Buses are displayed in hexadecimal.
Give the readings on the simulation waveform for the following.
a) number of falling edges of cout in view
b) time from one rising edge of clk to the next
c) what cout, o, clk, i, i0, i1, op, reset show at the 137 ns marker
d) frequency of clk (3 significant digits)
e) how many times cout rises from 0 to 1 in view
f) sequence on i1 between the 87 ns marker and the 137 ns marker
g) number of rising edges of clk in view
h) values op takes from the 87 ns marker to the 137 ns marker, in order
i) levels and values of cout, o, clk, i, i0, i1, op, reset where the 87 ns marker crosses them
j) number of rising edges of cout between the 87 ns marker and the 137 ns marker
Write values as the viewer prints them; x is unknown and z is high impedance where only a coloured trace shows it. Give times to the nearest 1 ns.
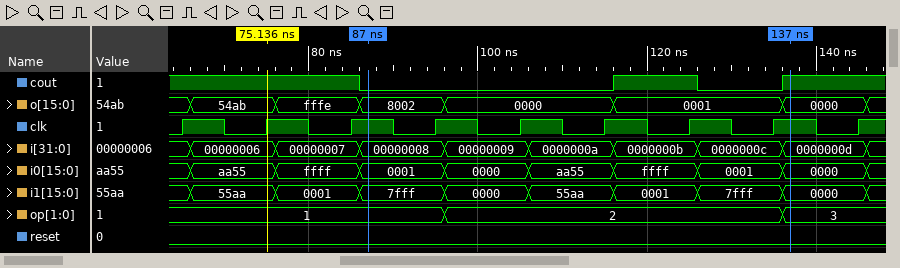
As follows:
2
10 ns
cout=1, o=0000, clk=1, i=0000000d, i0=0000, i1=0000, op=3, reset=0
100 MHz
2
7fff, 0000, 55aa, 0001, 7fff, 0000
9
1, 2, 3
cout=0, o=8002, clk=1, i=00000008, i0=0001, i1=7fff, op=1, reset=0
2
